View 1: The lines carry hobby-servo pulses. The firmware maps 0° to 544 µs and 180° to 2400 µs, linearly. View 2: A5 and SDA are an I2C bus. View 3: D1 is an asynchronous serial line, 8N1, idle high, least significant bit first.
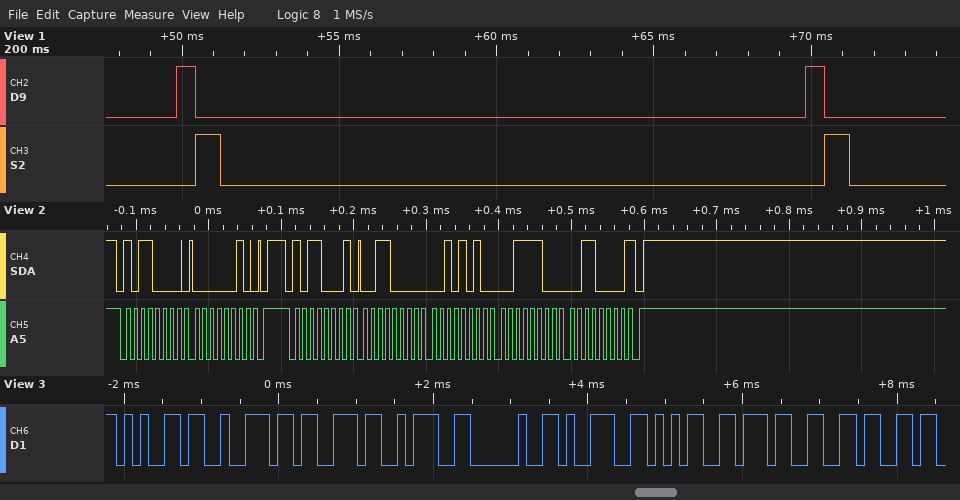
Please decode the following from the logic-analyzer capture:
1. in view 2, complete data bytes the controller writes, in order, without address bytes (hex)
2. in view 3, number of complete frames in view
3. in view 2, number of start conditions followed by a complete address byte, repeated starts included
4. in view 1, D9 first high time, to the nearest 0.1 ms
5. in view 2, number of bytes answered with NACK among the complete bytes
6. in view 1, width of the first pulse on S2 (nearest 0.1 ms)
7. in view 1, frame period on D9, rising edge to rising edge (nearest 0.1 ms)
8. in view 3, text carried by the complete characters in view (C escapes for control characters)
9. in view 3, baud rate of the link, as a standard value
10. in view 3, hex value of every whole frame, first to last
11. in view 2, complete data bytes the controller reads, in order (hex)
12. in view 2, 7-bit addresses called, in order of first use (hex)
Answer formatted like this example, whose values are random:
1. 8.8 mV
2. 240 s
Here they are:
1. 02
2. 9
3. 2
4. 0.6 ms
5. 1
6. 0.8 ms
7. 20.0 ms
8. "ers: 9576"
9. 9600 baud
10. 65 72 73 3A 20 39 35 37 36
11. 30 2A 3C 30
12. 0x58
